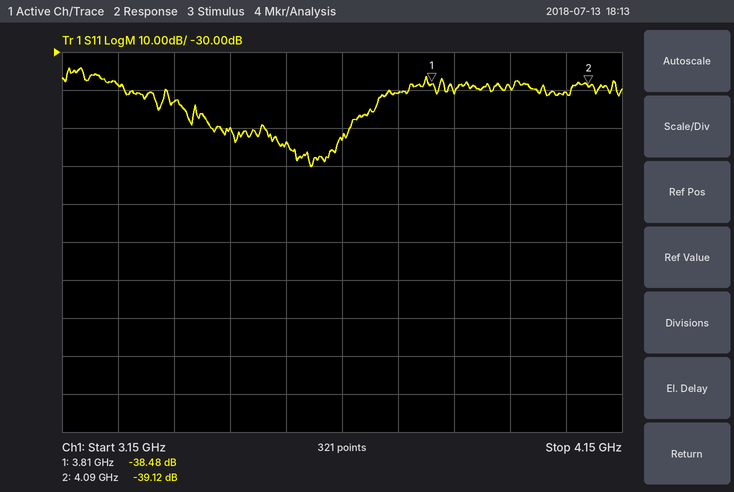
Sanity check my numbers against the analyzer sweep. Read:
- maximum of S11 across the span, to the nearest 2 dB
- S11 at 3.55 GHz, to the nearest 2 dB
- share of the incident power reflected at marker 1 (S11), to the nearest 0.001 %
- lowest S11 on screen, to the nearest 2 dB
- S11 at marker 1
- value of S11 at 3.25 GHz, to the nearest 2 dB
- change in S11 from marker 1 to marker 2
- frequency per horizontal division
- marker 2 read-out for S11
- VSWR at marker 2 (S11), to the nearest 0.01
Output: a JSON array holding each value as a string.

["-34 dB", "-54 dB", "0.014 %", "-60 dB", "-38.48 dB", "-38 dB", "-0.64 dB", "100 MHz", "-39.12 dB", "1.02"]
